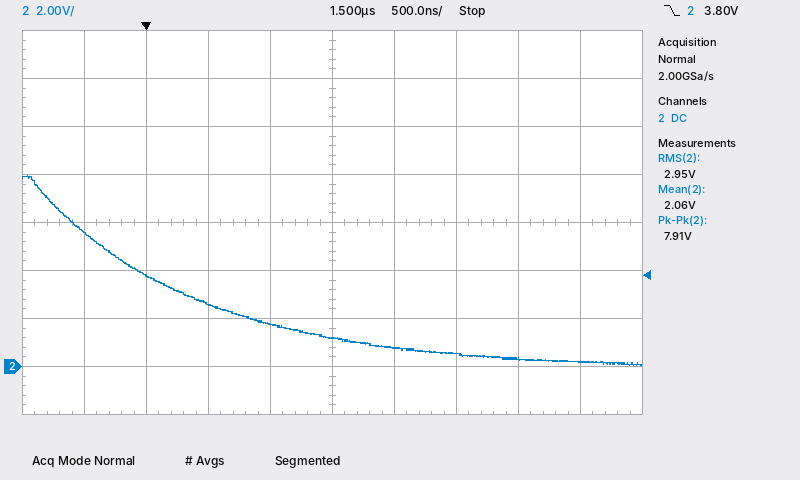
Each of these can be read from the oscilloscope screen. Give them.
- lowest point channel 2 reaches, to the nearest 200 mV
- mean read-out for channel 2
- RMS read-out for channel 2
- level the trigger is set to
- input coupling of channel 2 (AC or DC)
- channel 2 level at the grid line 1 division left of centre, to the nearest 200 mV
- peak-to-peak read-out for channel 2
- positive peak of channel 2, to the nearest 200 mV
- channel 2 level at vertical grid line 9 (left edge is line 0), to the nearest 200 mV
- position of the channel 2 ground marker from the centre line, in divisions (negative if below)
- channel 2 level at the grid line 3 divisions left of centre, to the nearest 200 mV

0.0 V
2.06 V
2.95 V
3.80 V
DC
1.8 V
7.91 V
8.0 V
200 mV
-3.0 div
3.8 V
